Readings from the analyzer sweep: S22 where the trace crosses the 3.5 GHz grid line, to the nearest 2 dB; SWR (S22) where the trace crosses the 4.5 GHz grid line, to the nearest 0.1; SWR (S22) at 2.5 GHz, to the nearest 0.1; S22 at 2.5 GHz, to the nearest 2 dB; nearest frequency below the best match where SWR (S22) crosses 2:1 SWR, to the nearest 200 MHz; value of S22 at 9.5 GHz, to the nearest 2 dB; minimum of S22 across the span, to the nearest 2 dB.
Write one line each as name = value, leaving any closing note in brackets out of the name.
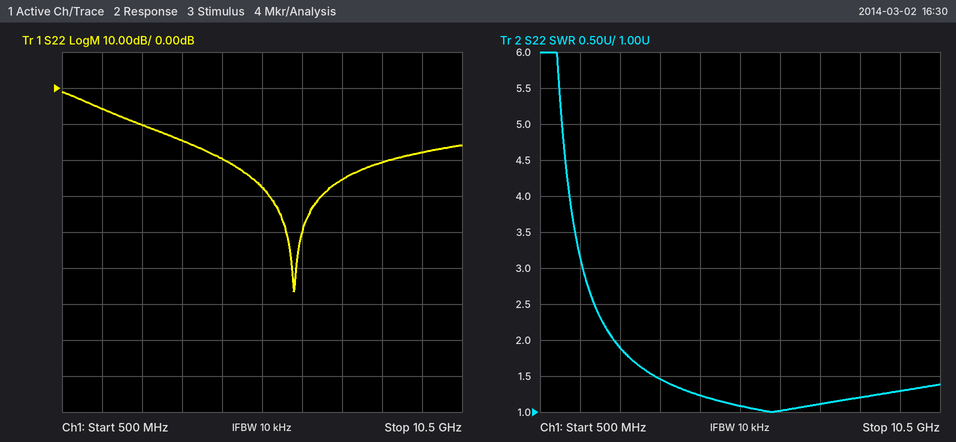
S22 where the trace crosses the 3.5 GHz grid line, to the nearest 2 dB = -14 dB
SWR (S22) where the trace crosses the 4.5 GHz grid line, to the nearest 0.1 = 1.2
SWR (S22) at 2.5 GHz, to the nearest 0.1 = 1.9
S22 at 2.5 GHz, to the nearest 2 dB = -10 dB
nearest frequency below the best match where SWR (S22) crosses 2:1 SWR, to the nearest 200 MHz = 2.4 GHz
value of S22 at 9.5 GHz, to the nearest 2 dB = -18 dB
minimum of S22 across the span, to the nearest 2 dB = -56 dB
